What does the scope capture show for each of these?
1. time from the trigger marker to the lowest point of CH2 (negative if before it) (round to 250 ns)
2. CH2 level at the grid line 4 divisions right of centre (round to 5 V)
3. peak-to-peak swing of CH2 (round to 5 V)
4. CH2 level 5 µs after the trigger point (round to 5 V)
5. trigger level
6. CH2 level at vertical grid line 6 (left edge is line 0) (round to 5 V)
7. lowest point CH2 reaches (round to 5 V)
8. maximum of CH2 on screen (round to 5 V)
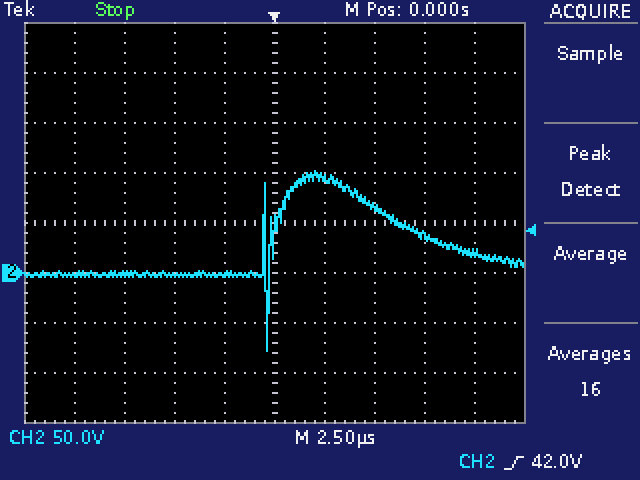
-250 ns
20 V
180 V
65 V
42.0 V
95 V
-80 V
100 V
